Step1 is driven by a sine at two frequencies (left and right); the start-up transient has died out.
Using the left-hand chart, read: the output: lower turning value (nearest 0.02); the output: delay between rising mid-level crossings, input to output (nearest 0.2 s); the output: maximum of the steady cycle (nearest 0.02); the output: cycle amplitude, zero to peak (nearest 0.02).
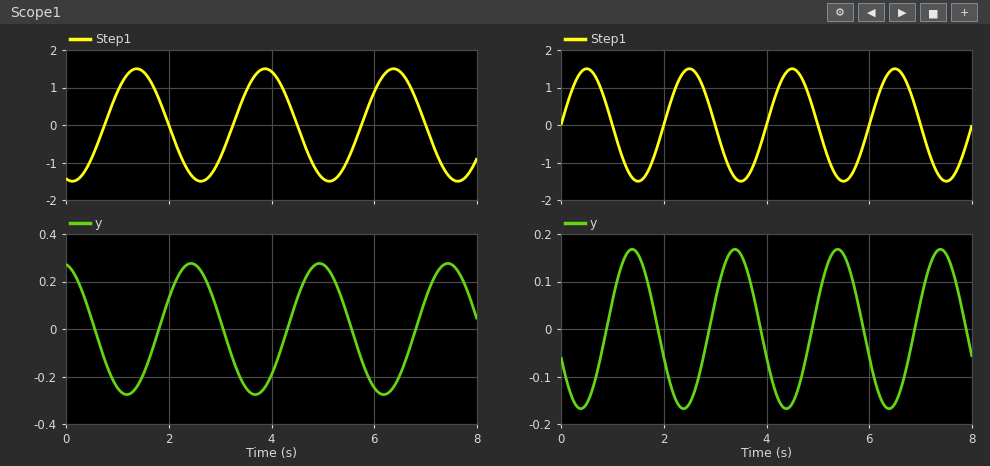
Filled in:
-0.28
1.0 s
0.28
0.28
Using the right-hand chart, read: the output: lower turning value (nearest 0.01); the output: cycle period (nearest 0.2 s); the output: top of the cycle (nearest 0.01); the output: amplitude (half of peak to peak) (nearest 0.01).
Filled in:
-0.17
2.0 s
0.17
0.17
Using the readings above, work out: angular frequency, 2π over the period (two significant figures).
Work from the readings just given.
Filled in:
3.1 rad/s
